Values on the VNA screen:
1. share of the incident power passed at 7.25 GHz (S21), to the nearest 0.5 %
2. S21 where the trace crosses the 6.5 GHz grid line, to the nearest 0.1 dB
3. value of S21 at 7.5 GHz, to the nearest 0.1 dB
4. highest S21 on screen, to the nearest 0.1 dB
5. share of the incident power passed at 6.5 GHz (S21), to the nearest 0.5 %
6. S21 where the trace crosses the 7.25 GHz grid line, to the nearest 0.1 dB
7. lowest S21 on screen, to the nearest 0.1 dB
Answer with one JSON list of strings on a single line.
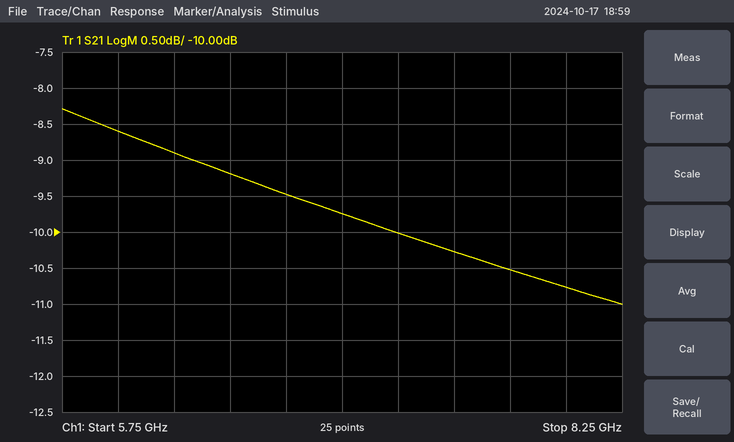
["10.0 %", "-9.2 dB", "-10.3 dB", "-8.3 dB", "12.0 %", "-10.0 dB", "-11.0 dB"]
